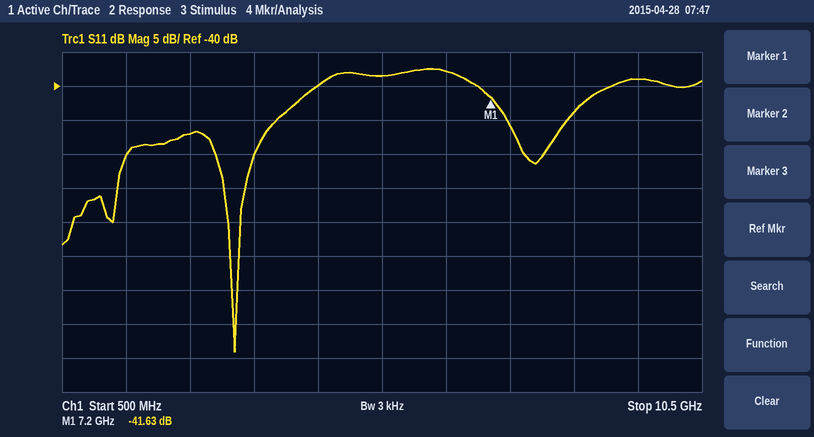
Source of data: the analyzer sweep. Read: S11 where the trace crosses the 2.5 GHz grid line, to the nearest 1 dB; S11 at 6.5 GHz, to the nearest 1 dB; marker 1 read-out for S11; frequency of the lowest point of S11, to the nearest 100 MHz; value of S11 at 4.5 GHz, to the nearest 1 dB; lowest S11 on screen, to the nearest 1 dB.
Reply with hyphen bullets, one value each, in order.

- -47 dB
- -38 dB
- -41.63 dB
- 3.2 GHz
- -40 dB
- -79 dB
